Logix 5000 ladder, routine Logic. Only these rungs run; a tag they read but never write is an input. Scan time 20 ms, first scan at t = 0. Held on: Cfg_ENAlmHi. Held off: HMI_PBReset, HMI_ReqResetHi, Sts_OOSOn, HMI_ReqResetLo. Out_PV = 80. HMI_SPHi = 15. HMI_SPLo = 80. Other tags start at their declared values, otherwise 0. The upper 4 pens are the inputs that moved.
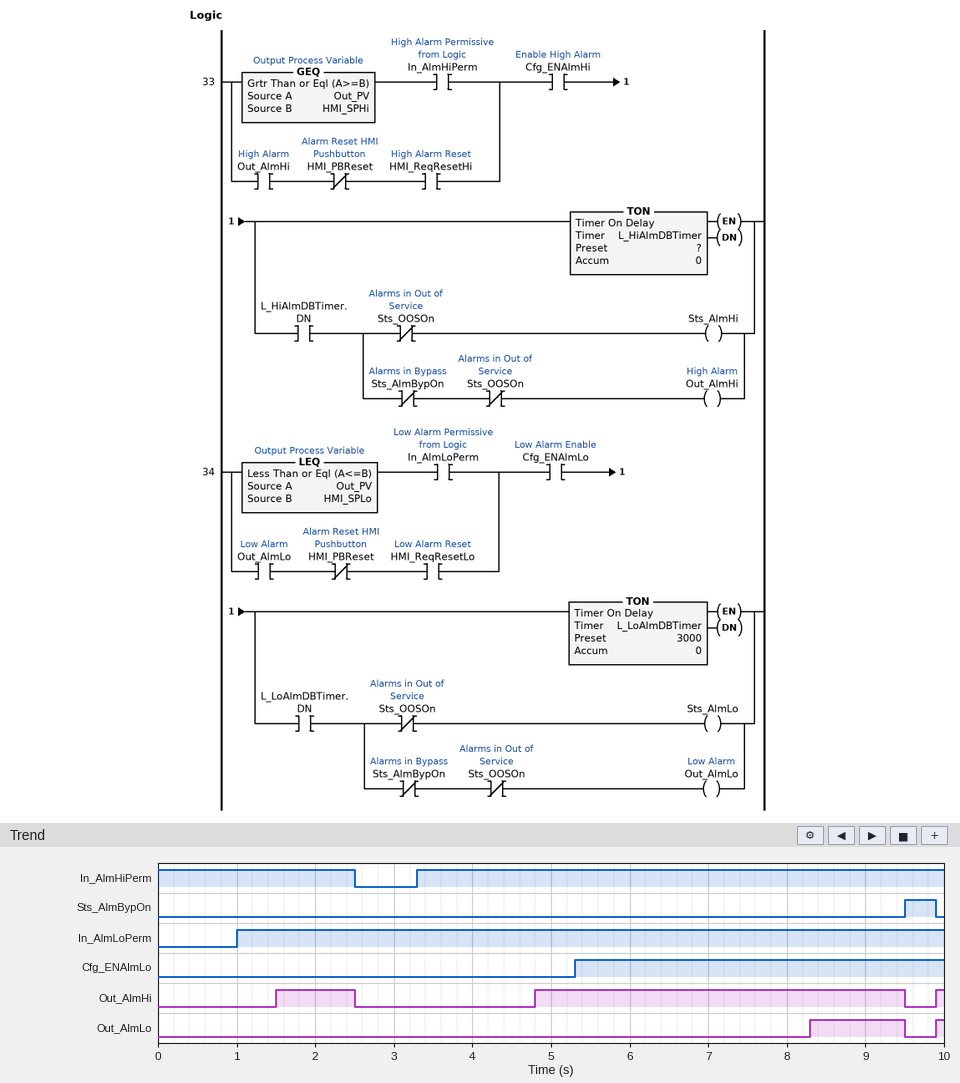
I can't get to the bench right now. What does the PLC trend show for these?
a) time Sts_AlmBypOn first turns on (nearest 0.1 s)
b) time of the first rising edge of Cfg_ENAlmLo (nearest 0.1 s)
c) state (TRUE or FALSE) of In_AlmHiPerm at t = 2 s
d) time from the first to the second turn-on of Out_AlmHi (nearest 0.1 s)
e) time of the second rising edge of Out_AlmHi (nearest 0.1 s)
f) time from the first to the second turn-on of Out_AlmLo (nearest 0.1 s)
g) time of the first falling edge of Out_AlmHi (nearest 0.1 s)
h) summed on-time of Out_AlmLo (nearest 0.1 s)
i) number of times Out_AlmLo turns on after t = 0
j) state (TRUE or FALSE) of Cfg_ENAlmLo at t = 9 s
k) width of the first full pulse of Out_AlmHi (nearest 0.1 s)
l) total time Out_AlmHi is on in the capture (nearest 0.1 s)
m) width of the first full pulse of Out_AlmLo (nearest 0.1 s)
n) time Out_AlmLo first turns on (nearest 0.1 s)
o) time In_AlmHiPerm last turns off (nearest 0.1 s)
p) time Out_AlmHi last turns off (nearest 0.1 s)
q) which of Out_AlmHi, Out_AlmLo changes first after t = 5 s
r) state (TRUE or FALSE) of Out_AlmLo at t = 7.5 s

9.5 s
5.3 s
TRUE
3.3 s
4.8 s
1.6 s
2.5 s
1.3 s
2
TRUE
1.0 s
5.8 s
1.2 s
8.3 s
2.5 s
9.5 s
Out_AlmLo
FALSE
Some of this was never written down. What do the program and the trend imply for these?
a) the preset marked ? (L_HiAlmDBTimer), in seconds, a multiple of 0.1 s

1.5 s
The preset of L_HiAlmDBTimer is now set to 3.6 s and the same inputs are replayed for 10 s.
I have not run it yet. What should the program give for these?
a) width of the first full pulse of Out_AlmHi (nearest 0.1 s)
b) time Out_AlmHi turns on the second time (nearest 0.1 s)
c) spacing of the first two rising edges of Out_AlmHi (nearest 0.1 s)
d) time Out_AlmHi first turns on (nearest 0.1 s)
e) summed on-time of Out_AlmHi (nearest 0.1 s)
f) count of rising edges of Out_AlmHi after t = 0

2.6 s
9.9 s
3.0 s
6.9 s
2.7 s
2
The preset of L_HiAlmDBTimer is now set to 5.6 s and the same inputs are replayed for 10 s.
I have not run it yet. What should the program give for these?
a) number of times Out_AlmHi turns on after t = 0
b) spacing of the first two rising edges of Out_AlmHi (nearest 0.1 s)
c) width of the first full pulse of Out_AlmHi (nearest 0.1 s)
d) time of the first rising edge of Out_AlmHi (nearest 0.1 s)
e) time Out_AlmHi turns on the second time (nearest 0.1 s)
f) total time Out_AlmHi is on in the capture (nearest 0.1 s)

2
1.0 s
0.6 s
8.9 s
9.9 s
0.7 s
